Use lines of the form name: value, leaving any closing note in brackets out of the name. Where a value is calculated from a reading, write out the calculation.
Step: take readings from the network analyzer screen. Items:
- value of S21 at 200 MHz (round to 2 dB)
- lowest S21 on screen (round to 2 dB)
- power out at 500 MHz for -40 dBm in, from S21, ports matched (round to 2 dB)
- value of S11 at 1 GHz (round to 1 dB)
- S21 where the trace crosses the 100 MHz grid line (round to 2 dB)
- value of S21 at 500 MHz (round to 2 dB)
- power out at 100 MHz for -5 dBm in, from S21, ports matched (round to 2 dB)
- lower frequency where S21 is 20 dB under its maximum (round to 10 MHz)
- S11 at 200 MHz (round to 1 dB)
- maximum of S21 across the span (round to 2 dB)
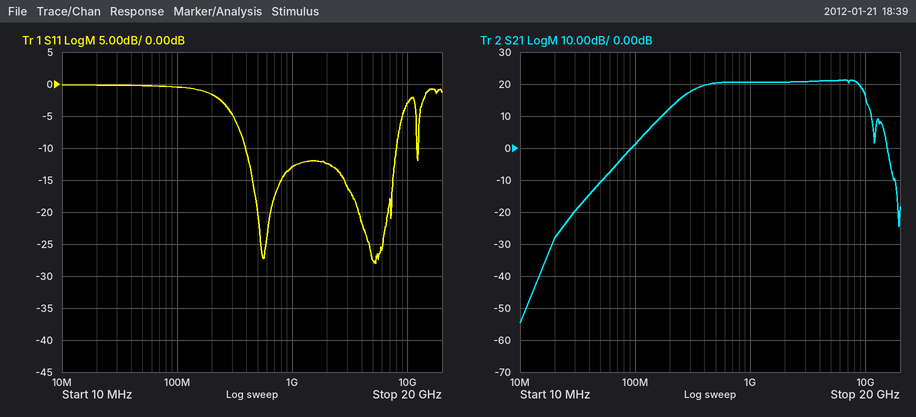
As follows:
value of S21 at 200 MHz: 12 dB
lowest S21 on screen: -54 dB
power out at 500 MHz for -40 dBm in, from S21, ports matched: -40 dBm + (20 dB) = -20 dBm
value of S11 at 1 GHz: -13 dB
S21 where the trace crosses the 100 MHz grid line: 2 dB
value of S21 at 500 MHz: 20 dB
power out at 100 MHz for -5 dBm in, from S21, ports matched: -5 dBm + (2 dB) = -4 dBm
lower frequency where S21 is 20 dB under its maximum: 100 MHz
S11 at 200 MHz: -2 dB
maximum of S21 across the span: 22 dB
